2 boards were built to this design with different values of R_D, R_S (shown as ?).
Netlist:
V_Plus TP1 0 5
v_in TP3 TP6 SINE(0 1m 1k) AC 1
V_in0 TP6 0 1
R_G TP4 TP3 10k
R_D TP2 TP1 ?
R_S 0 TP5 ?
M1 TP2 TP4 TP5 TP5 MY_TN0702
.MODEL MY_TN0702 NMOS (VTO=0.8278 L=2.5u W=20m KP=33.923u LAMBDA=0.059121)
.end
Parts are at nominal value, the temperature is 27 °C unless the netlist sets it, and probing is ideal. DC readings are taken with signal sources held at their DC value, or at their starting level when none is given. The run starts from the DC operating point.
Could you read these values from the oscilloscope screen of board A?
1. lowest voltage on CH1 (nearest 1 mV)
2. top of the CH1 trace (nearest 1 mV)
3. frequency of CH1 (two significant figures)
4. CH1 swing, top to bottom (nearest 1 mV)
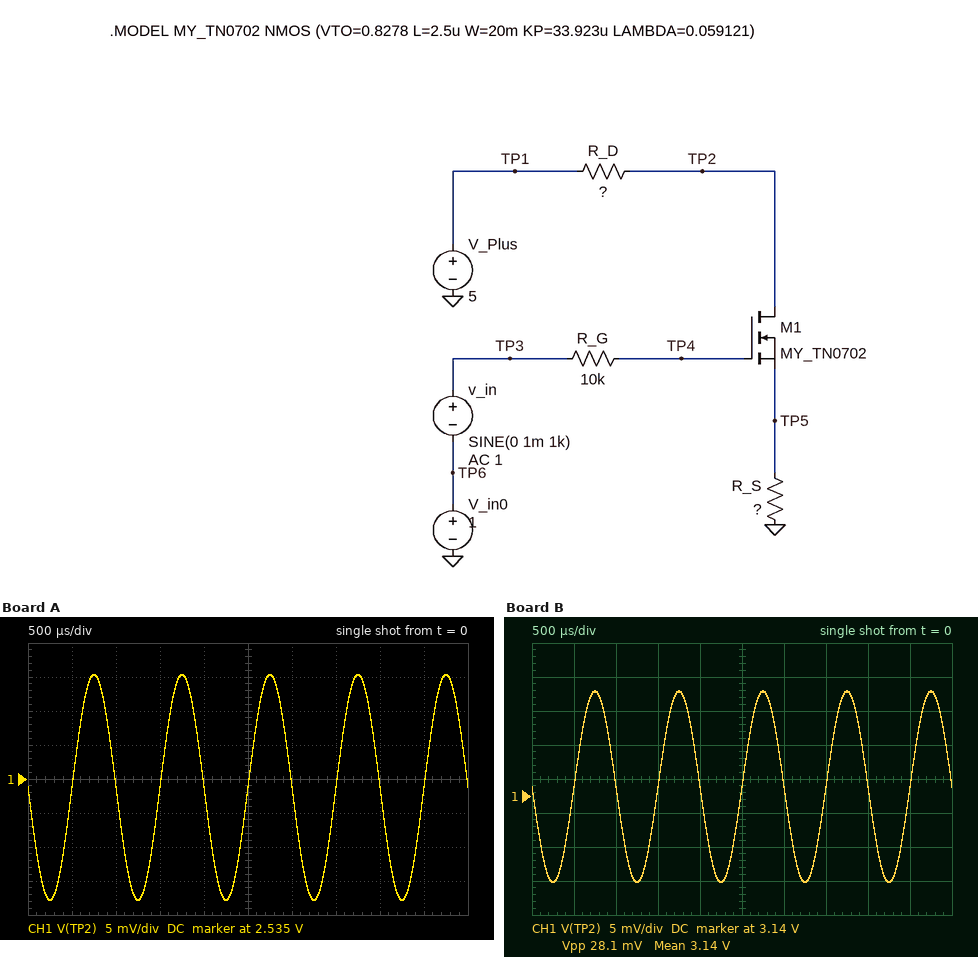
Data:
2.517 V
2.550 V
1.0 kHz
33 mV
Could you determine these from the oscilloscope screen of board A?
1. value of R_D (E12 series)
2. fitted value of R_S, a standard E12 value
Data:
5.6 kΩ
270 Ω
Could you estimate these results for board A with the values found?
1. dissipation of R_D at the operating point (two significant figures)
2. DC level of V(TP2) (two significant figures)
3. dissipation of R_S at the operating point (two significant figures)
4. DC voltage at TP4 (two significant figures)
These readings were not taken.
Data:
1.1 mW
2.5 V
52 µW
1.0 V
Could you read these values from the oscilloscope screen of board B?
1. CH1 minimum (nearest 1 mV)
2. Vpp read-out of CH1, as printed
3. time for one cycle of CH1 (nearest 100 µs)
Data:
3.127 V
28.1 mV
1.0 ms
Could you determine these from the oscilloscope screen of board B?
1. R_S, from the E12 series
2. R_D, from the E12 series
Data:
68 Ω
1.5 kΩ
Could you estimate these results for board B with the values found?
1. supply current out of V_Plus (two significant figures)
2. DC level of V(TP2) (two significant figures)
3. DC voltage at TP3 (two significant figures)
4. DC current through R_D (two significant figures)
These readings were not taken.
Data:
1.2 mA
3.1 V
1.0 V
1.2 mA
